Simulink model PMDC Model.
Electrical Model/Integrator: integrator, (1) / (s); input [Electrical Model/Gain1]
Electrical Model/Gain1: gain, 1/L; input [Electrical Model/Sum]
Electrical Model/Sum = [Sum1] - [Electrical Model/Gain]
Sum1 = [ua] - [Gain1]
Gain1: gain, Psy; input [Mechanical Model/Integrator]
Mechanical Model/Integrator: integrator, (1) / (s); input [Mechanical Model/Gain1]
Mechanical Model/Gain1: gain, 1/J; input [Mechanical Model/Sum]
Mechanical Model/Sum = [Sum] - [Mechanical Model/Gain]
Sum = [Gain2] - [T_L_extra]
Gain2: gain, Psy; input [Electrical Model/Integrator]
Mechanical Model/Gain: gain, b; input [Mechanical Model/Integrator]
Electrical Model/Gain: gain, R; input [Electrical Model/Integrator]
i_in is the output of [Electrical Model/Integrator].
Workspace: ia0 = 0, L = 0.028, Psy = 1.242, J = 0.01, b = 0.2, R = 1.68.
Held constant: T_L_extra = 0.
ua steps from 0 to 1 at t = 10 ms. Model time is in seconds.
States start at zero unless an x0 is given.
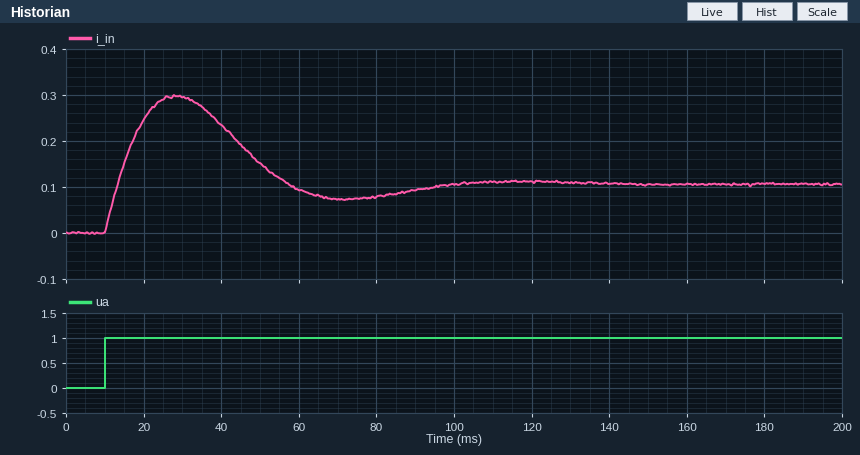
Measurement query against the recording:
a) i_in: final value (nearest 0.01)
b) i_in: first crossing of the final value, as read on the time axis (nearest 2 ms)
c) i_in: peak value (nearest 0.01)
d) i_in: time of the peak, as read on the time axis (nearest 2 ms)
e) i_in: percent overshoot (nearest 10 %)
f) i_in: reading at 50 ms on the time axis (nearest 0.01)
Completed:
0.11
14 ms
0.30
28 ms
180 %
0.15
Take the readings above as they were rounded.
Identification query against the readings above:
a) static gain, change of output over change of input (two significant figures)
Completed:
0.11
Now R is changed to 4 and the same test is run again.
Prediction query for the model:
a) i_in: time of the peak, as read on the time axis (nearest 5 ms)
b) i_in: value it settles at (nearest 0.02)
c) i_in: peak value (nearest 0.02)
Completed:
25 ms
0.08
0.18
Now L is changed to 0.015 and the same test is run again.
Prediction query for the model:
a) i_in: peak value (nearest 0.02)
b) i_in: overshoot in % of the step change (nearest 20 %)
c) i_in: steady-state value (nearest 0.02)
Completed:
0.34
220 %
0.10
